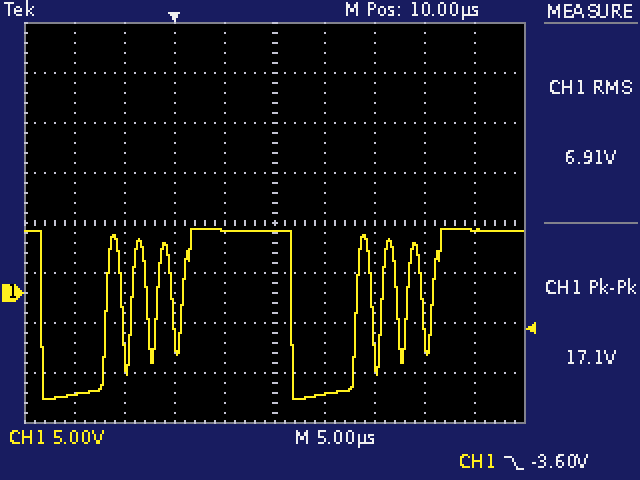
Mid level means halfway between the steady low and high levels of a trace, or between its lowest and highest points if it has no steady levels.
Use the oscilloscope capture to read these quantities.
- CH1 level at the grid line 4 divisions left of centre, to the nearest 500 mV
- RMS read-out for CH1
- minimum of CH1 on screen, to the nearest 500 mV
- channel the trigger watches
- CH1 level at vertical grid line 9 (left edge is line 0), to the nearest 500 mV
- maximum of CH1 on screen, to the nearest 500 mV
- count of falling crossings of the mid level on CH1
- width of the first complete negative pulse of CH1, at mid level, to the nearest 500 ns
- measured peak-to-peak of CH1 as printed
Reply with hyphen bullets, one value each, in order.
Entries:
- -10.0 V
- 6.91 V
- -10.5 V
- CH1
- 6.5 V
- 6.5 V
- 8
- 6.5 µs
- 17.1 V
